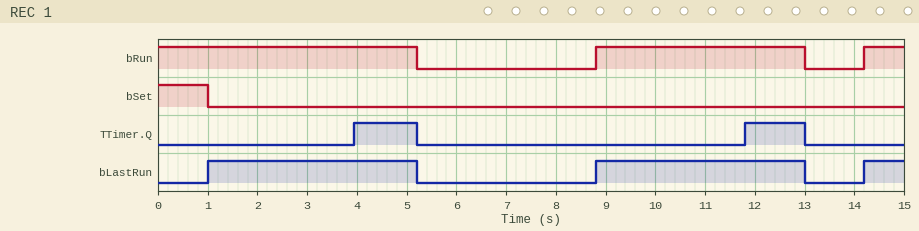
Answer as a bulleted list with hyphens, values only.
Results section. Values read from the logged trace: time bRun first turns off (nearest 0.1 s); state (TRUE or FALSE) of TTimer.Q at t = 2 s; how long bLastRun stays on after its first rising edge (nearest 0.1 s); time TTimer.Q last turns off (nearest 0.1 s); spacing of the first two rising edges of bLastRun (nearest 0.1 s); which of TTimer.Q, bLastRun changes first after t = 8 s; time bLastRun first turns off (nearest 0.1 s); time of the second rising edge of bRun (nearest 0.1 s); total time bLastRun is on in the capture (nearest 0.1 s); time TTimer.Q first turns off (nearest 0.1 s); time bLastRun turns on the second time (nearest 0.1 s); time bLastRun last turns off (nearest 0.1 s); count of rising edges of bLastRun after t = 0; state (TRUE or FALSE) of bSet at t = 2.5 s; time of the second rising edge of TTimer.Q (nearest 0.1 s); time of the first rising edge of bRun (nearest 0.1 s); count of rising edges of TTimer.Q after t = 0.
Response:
- 5.2 s
- FALSE
- 4.2 s
- 13.0 s
- 7.8 s
- bLastRun
- 5.2 s
- 14.2 s
- 9.2 s
- 5.2 s
- 8.8 s
- 13.0 s
- 3
- FALSE
- 11.8 s
- 8.8 s
- 2
